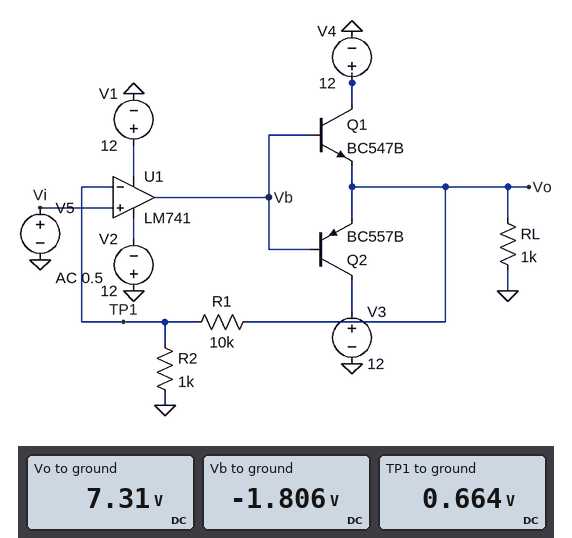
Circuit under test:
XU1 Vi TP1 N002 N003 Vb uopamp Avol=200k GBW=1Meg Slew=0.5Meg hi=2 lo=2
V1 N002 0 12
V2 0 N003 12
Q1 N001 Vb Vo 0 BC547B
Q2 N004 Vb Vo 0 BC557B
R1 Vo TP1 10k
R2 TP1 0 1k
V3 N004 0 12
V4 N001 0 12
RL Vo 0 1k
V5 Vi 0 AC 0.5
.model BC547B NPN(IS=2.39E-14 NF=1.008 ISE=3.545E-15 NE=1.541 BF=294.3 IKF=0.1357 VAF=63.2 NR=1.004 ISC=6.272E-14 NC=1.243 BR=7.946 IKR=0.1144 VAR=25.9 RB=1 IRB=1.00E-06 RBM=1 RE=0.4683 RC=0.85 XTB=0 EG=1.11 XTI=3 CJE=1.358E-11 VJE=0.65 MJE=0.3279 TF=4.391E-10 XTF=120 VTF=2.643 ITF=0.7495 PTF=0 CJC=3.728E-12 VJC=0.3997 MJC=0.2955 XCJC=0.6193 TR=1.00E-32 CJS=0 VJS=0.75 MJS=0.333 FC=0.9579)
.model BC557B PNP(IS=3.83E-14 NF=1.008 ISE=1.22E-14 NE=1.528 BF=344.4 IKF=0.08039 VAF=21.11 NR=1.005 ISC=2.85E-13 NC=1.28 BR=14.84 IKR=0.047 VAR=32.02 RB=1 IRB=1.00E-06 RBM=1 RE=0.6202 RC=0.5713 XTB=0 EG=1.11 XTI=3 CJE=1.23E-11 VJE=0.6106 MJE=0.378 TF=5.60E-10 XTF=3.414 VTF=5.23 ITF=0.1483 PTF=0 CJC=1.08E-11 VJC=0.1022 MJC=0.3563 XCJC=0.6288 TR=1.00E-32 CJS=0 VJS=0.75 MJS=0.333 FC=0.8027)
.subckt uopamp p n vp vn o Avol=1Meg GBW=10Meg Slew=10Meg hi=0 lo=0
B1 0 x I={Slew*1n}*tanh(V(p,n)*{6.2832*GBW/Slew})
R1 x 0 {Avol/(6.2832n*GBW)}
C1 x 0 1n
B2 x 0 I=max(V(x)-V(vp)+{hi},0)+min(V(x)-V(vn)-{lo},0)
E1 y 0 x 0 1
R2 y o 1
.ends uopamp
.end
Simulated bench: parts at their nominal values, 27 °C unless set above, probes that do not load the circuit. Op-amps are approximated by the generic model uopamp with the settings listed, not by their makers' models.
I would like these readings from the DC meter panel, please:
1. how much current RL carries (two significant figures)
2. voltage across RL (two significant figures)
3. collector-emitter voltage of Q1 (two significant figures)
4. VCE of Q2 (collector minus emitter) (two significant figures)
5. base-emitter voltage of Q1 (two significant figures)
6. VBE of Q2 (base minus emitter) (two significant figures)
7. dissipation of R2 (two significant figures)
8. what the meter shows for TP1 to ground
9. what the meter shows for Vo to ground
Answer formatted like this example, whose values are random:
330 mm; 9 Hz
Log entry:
7.3 mA; 7.3 V; 4.7 V; 4.7 V; -9.1 V; -9.1 V; 440 µW; 0.664 V; 7.31 V
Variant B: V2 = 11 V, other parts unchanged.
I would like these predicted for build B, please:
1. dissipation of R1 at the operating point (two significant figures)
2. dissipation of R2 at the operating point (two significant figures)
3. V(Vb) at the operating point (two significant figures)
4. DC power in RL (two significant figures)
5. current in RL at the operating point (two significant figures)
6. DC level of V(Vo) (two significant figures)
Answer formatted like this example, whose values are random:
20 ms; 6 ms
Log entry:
4.7 mW; 470 µW; -1.2 V; 57 mW; 7.5 mA; 7.5 V
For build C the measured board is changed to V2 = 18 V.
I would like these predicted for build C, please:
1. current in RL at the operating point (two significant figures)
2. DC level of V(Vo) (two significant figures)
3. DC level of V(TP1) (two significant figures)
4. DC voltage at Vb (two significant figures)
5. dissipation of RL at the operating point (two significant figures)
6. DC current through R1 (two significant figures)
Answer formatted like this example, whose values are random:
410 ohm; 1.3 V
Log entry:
6.0 mA; 6.0 V; 540 mV; -5.5 V; 36 mW; 540 µA
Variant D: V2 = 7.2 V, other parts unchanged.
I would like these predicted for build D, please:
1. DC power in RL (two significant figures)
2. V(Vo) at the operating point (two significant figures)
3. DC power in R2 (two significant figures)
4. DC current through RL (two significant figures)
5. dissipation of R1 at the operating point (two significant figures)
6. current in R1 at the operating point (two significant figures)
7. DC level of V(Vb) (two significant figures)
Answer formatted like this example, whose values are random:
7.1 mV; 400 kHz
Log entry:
70 mW; 8.4 V; 580 µW; 8.4 mA; 5.8 mW; 760 µA; 1.1 V
